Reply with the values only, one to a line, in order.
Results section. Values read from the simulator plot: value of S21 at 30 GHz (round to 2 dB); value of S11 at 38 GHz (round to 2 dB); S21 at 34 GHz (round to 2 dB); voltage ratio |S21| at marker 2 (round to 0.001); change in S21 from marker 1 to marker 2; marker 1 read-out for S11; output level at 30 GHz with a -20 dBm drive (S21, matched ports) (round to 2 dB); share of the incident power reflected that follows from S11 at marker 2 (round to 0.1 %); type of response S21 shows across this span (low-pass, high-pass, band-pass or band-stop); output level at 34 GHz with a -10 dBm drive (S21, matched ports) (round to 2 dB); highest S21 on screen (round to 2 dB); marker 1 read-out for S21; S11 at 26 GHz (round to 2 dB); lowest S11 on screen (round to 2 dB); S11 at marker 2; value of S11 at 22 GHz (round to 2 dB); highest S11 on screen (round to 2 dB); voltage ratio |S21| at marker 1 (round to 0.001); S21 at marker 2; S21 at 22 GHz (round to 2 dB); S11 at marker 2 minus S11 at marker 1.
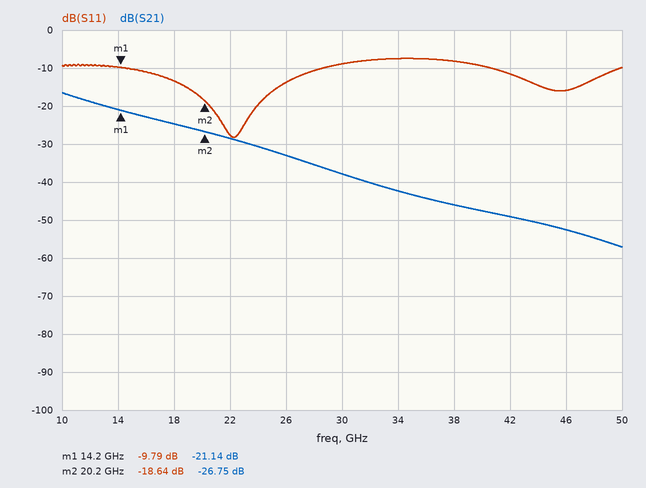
-38 dB
-8 dB
-42 dB
0.046
-5.61 dB
-9.79 dB
-58 dBm
1.4 %
low-pass
-52 dBm
-16 dB
-21.14 dB
-14 dB
-28 dB
-18.64 dB
-28 dB
-8 dB
0.088
-26.75 dB
-28 dB
-8.85 dB
